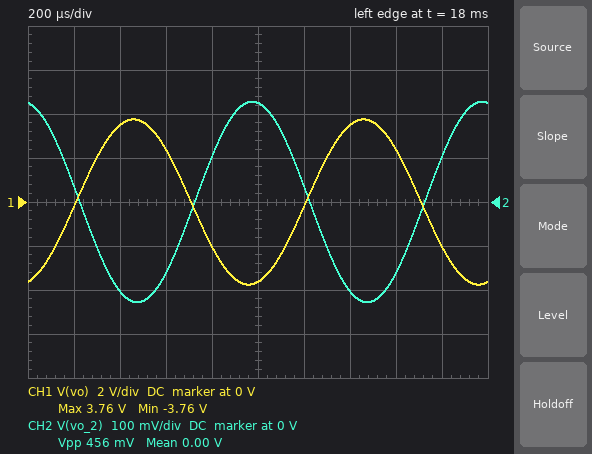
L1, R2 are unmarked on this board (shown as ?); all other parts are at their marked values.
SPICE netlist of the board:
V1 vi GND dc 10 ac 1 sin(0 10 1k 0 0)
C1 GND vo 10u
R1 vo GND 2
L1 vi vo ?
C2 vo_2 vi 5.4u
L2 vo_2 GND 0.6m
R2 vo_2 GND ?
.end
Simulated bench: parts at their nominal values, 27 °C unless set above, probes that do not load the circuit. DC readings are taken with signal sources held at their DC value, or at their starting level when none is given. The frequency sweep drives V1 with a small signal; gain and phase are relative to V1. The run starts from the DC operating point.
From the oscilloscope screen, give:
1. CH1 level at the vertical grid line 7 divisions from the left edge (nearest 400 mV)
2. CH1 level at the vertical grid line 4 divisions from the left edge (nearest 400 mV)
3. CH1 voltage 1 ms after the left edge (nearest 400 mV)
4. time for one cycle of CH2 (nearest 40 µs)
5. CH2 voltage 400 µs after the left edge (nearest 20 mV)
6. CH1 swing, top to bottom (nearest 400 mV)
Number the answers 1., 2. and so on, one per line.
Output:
1. 3.6 V
2. -2.0 V
3. -3.6 V
4. 1.00 ms
5. -200 mV
6. 7.6 V
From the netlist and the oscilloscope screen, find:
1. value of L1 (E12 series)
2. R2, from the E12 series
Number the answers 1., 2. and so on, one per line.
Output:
1. 820 µH
2. 0.68 Ω
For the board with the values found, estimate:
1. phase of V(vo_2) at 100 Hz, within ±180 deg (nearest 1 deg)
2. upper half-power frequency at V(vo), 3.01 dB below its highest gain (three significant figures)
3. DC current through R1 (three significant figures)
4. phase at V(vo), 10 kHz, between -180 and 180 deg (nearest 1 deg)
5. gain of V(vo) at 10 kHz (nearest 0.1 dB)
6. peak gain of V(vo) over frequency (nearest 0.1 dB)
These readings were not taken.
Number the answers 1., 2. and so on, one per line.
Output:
1. 151 deg
2. 408 Hz
3. 5.00 A
4. -141 deg
5. -32.2 dB
6. 0 dB
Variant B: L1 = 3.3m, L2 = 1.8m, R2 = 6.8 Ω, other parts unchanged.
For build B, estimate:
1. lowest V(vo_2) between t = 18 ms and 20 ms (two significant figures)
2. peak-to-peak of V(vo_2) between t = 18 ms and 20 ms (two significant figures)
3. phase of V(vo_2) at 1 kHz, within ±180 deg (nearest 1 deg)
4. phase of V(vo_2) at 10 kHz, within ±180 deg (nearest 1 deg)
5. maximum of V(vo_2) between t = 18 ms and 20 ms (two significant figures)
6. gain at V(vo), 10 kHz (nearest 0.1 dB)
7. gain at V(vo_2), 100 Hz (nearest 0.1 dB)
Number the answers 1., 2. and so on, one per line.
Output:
1. -2.2 V
2. 4.3 V
3. 110 deg
4. 24 deg
5. 2.2 V
6. -44.4 dB
7. -48.4 dB
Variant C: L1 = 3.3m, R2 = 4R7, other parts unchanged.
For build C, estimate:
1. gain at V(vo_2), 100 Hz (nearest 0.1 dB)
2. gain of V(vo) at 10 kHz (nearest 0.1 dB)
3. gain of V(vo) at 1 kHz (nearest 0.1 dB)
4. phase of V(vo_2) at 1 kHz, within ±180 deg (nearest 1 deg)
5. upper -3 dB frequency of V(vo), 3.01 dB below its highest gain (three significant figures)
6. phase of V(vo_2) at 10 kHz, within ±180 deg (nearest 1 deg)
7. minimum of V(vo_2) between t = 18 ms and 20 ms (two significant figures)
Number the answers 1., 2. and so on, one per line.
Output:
1. -57.9 dB
2. -44.4 dB
3. -20.3 dB
4. 137 deg
5. 97.6 Hz
6. 34 deg
7. -1.1 V
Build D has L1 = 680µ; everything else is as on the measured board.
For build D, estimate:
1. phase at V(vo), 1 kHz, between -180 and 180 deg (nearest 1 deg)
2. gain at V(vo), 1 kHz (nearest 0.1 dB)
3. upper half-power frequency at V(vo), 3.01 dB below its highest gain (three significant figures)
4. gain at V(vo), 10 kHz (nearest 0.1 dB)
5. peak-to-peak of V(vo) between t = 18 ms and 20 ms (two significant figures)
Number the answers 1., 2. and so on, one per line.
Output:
1. -71 deg
2. -7.1 dB
3. 497 Hz
4. -30.5 dB
5. 8.9 V
